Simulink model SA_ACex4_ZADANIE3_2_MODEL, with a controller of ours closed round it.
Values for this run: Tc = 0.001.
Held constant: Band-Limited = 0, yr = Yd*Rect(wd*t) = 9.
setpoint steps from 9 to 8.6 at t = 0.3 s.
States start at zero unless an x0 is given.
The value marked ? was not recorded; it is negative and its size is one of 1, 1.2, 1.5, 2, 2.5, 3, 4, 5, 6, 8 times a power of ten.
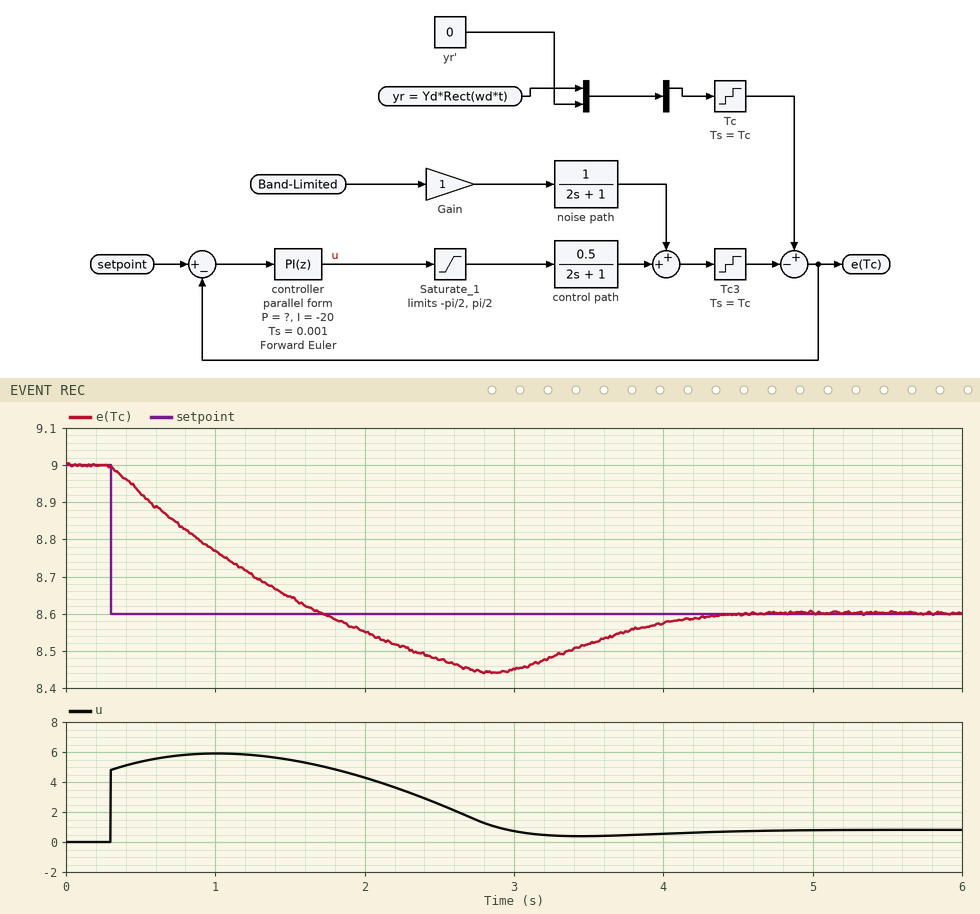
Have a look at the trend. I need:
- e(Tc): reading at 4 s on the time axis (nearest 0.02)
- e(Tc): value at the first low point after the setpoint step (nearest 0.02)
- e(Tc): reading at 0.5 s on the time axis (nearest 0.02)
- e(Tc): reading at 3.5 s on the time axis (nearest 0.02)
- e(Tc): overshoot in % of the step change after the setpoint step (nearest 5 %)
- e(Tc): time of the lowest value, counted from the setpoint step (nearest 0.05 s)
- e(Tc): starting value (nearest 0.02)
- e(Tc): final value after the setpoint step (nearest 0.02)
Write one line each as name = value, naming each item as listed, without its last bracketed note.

e(Tc): reading at 4 s on the time axis = 8.58
e(Tc): value at the first low point after the setpoint step = 8.44
e(Tc): reading at 0.5 s on the time axis = 8.92
e(Tc): reading at 3.5 s on the time axis = 8.52
e(Tc): overshoot in % of the step change after the setpoint step = 40 %
e(Tc): time of the lowest value, counted from the setpoint step = 2.55 s
e(Tc): starting value = 9.00
e(Tc): final value after the setpoint step = 8.60
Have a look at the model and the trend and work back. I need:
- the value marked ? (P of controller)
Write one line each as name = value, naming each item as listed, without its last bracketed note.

the value marked ? = -12
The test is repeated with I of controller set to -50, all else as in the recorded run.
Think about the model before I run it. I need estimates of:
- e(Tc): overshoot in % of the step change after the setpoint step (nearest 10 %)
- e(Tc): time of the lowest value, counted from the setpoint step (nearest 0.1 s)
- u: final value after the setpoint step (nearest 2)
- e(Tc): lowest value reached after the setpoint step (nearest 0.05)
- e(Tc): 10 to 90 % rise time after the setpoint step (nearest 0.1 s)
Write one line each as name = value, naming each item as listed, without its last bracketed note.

e(Tc): overshoot in % of the step change after the setpoint step = 50 %
e(Tc): time of the lowest value, counted from the setpoint step = 3.0 s
u: final value after the setpoint step = 0
e(Tc): lowest value reached after the setpoint step = 8.40
e(Tc): 10 to 90 % rise time after the setpoint step = 1.1 s
